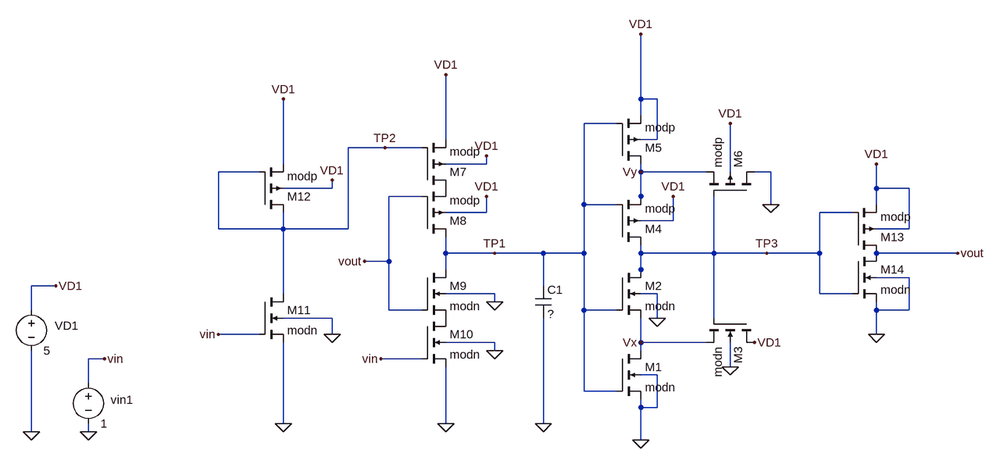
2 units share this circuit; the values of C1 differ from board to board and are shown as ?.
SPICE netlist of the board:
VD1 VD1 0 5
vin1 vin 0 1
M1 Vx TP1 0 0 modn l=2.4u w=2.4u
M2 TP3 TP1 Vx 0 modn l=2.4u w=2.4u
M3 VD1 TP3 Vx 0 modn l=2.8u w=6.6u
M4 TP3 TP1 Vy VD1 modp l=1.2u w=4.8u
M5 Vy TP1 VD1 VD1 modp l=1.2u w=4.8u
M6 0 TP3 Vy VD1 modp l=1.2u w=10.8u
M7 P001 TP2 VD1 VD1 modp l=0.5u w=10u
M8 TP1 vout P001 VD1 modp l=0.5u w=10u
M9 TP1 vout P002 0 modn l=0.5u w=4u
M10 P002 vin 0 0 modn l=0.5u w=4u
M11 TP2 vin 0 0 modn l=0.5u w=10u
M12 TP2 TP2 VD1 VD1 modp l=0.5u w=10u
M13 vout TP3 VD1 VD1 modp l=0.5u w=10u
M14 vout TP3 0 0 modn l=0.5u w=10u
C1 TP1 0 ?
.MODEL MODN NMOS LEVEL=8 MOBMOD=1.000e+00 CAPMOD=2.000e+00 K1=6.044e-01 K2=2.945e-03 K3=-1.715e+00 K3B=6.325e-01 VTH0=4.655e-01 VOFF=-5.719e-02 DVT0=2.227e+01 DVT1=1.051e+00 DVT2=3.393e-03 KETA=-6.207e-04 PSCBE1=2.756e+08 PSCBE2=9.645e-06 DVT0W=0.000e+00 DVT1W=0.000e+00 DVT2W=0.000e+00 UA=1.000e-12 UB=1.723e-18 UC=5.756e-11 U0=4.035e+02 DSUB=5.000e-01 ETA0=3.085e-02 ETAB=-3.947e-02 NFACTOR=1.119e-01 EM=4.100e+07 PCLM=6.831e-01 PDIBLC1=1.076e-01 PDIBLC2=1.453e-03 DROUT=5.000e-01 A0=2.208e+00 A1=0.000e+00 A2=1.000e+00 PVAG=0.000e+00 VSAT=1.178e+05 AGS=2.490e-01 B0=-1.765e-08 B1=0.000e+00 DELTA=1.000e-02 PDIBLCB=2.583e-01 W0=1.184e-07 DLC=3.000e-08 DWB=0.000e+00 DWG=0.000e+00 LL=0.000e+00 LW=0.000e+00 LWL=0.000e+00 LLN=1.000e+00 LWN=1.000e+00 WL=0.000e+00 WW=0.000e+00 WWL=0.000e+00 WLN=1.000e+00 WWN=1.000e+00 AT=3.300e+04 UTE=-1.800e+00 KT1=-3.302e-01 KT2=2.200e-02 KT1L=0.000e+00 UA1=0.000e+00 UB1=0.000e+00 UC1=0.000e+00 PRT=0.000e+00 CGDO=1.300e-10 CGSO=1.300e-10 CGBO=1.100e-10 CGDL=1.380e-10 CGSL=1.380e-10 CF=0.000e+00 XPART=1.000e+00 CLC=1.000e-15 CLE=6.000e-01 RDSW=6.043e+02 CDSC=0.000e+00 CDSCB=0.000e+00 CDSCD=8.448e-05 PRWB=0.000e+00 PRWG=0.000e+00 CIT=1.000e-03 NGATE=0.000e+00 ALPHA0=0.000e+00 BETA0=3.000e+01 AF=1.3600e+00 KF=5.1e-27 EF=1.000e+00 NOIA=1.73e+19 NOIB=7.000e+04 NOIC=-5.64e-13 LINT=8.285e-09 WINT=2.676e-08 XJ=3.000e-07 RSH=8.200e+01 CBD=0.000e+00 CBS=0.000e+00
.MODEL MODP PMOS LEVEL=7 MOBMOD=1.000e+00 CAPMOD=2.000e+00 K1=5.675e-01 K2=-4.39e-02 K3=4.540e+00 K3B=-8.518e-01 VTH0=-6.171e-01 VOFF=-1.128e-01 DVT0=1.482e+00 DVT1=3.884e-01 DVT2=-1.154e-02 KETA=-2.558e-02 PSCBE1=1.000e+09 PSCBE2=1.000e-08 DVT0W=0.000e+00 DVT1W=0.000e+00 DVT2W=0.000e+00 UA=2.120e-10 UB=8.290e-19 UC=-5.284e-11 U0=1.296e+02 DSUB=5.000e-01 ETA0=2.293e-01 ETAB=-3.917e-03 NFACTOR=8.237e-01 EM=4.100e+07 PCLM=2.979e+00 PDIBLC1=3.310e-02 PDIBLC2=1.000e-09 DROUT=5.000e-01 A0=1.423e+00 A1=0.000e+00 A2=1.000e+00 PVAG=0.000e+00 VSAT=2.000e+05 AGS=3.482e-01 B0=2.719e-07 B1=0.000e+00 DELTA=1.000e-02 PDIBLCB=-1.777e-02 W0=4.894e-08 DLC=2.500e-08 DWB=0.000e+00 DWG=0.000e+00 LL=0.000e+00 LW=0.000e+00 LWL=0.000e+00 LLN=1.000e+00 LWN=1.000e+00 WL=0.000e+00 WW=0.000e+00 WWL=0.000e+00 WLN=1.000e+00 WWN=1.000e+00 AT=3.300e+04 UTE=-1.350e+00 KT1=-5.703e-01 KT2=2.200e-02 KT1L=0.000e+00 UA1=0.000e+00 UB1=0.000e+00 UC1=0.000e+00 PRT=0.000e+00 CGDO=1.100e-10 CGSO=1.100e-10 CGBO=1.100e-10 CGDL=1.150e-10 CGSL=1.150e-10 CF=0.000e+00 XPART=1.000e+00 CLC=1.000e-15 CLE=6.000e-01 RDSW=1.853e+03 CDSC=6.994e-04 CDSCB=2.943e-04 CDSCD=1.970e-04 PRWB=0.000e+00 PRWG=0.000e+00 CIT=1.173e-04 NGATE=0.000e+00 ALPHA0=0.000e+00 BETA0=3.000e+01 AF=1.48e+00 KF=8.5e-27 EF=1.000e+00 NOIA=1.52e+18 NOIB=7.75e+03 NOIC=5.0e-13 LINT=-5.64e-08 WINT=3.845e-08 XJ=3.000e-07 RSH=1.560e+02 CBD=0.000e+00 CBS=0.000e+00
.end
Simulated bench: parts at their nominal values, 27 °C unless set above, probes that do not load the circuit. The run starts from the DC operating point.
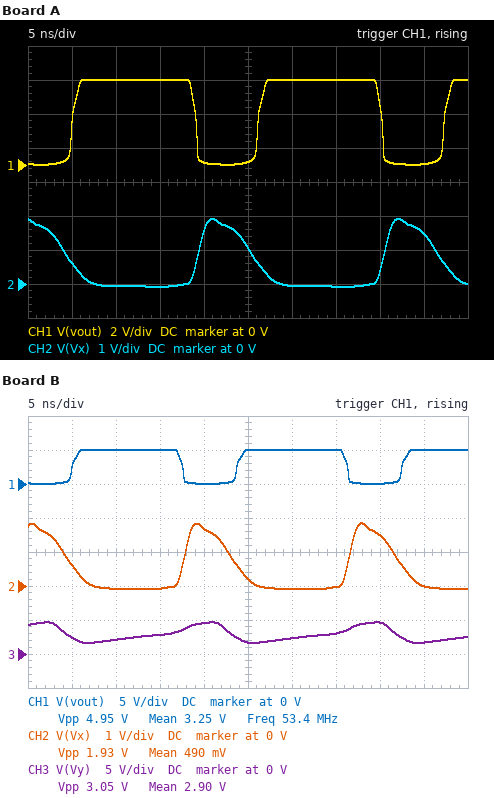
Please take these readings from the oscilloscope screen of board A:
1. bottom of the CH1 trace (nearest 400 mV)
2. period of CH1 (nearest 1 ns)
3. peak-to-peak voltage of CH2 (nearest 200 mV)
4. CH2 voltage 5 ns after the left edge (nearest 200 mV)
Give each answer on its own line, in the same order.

0 V
21 ns
2.0 V
600 mV
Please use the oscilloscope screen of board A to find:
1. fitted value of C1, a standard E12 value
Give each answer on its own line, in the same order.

560 fF
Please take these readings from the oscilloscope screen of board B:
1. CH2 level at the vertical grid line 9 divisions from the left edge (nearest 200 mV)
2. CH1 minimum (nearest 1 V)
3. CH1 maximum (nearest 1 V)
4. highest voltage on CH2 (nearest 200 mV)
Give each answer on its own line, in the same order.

0 V
0 V
5 V
1.8 V
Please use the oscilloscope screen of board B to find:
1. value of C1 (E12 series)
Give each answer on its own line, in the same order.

470 fF
